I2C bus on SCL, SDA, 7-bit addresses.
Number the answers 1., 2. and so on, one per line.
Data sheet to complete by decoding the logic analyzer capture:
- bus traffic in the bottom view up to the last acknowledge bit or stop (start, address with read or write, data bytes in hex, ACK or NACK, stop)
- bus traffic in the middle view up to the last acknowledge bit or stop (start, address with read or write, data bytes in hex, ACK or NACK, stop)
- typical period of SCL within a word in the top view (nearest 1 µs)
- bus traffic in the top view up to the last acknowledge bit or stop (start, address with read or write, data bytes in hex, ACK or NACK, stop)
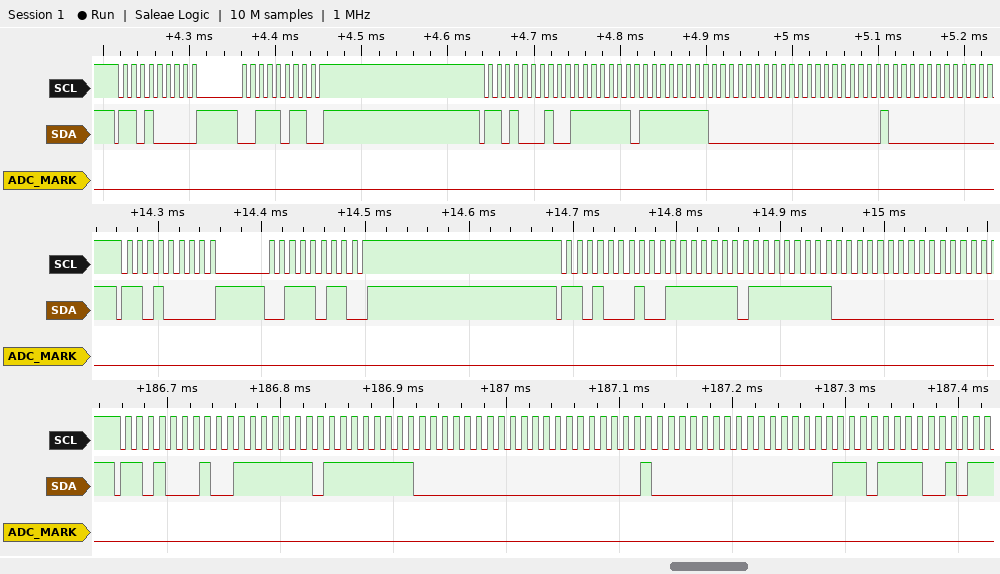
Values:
1. start, address 68 read ACK, 7F ACK, FF ACK, 00 ACK, 00 ACK, 40 ACK, 00 ACK, EF ACK
2. start, address 68 write ACK, 3B ACK, stop, start, address 68 read ACK, 7F ACK, FF ACK, 00 ACK
3. 10 µs
4. start, address 68 write ACK, 3B ACK, stop, start, address 68 read ACK, 7F ACK, FF ACK, 00 ACK, 00 ACK, 40 ACK
